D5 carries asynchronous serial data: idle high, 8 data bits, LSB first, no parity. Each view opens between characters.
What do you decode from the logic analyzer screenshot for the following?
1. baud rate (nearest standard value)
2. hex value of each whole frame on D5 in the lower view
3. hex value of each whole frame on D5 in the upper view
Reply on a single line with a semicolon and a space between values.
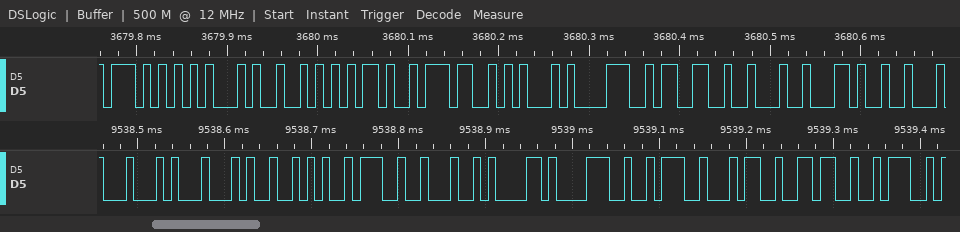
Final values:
115200 baud; 44, 44, 52, 3A, 22, 61, 38, 3A, 34, 36, 3A; 57, 45, 52, 2D, 37, 45, 38, 33, 22, 2C
